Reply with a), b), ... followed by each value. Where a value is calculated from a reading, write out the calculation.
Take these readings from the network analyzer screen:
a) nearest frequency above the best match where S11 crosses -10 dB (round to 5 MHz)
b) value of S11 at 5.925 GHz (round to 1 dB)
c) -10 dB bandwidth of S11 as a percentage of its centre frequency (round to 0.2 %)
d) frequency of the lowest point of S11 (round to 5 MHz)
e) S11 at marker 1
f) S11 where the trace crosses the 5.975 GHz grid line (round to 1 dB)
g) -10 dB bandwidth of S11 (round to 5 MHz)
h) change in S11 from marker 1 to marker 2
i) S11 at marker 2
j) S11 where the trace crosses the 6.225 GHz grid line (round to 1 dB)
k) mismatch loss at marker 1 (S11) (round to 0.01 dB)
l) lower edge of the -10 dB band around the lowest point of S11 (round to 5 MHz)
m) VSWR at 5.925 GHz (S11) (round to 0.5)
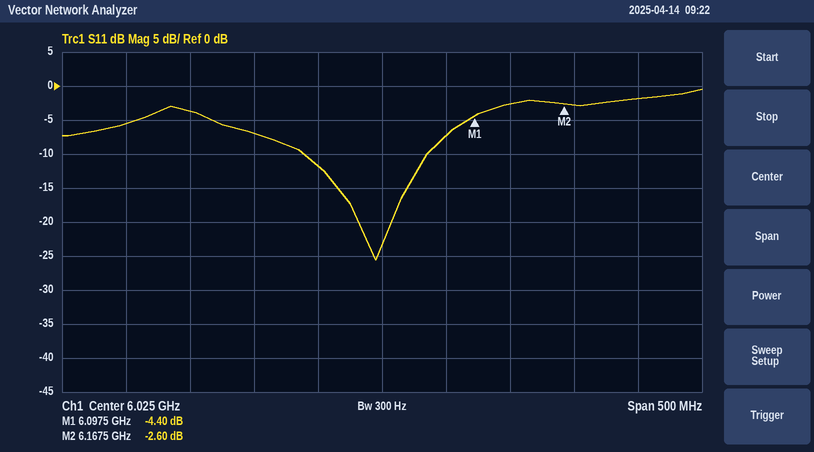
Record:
a) 6.060 GHz
b) -7 dB
c) 95 MHz / 6.0125 GHz ≈ 1.6 %
d) 6.020 GHz
e) -4.40 dB
f) -12 dB
g) 6.060 GHz − 5.965 GHz = 95 MHz
h) -2.6 − (-4.4) = 1.80 dB
i) -2.60 dB
j) -2 dB
k) −10 log10(1 − 10^(-4.4/10)) ≈ 1.96 dB
l) 5.965 GHz
m) |Γ| = 10^(-7/20) = 0.4467; VSWR = (1 + 0.4467)/(1 − 0.4467) ≈ 2.61, so 2.5 to the nearest 0.5
